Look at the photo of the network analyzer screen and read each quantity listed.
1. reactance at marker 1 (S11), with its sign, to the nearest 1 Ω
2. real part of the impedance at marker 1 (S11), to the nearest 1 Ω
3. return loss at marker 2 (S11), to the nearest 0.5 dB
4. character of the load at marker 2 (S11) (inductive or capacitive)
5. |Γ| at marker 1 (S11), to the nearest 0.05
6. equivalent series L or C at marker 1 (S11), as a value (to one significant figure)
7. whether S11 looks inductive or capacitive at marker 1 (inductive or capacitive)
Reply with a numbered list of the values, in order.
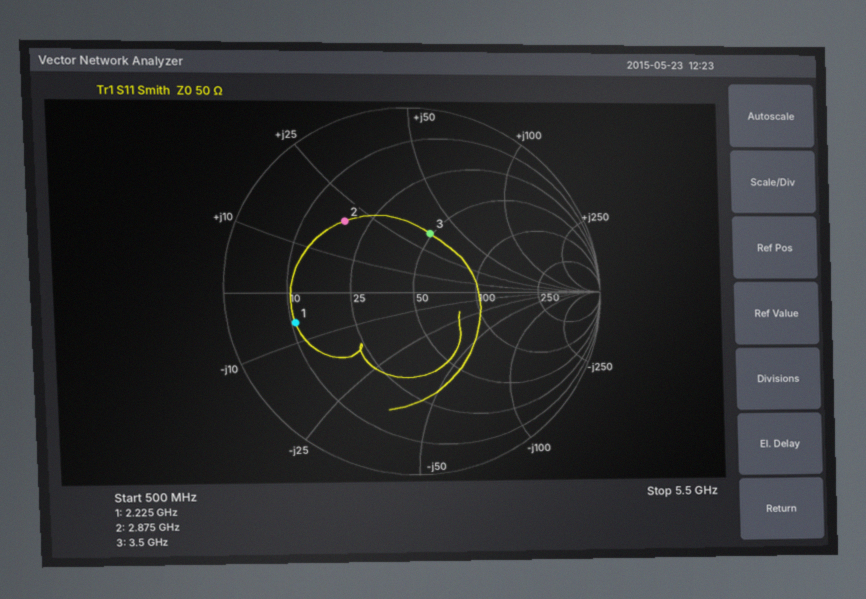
1. -6 Ω
2. 11 Ω
3. 5.5 dB
4. inductive
5. 0.65
6. 10 pF
7. capacitive
